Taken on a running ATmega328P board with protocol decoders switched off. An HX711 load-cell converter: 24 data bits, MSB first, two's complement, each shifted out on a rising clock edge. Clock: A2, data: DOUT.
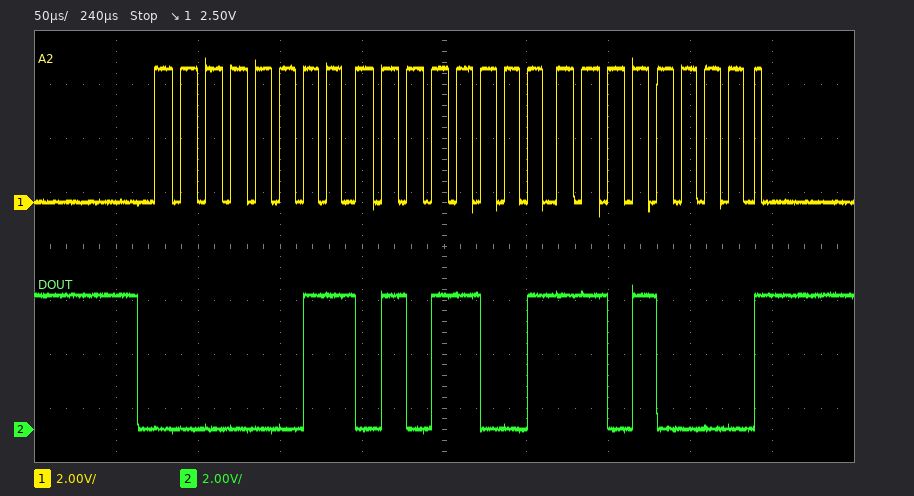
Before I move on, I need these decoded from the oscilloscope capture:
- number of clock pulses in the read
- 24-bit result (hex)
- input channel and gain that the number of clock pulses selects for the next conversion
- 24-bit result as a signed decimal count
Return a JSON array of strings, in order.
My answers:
["25", "0x0359D0", "channel A, gain 128", "219600"]
